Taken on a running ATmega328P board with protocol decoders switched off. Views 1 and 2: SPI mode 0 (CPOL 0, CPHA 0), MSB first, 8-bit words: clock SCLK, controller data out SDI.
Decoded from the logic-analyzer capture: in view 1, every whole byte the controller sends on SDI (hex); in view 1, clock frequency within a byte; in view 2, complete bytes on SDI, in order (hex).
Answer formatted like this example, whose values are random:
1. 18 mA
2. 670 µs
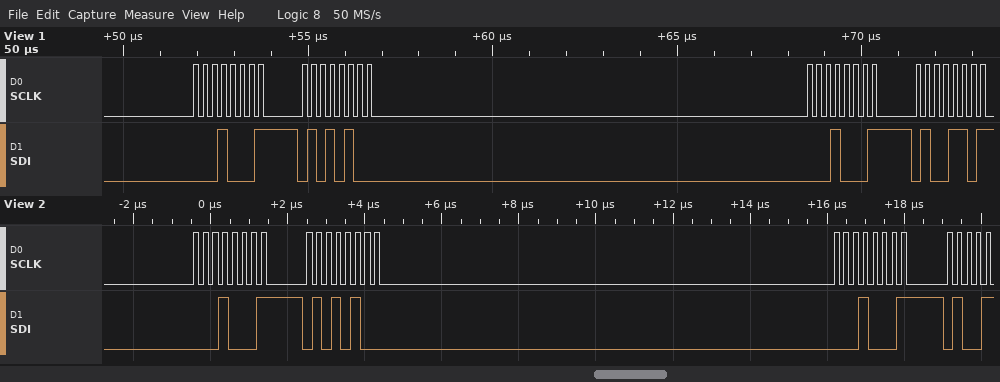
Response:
1. 11 54 11 4D
2. 4 MHz
3. 11 54 11
